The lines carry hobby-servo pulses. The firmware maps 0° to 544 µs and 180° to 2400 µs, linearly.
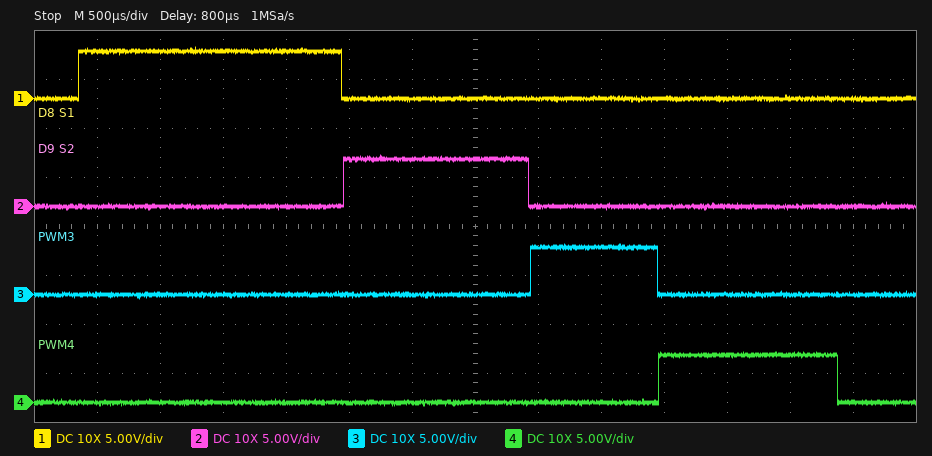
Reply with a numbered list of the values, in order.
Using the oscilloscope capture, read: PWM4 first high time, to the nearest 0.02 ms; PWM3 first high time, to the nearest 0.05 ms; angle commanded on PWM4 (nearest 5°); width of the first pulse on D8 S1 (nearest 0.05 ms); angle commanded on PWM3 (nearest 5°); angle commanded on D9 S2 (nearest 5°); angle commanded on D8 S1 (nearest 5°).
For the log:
1. 1.42 ms
2. 1.00 ms
3. 85°
4. 2.10 ms
5. 45°
6. 90°
7. 150°
